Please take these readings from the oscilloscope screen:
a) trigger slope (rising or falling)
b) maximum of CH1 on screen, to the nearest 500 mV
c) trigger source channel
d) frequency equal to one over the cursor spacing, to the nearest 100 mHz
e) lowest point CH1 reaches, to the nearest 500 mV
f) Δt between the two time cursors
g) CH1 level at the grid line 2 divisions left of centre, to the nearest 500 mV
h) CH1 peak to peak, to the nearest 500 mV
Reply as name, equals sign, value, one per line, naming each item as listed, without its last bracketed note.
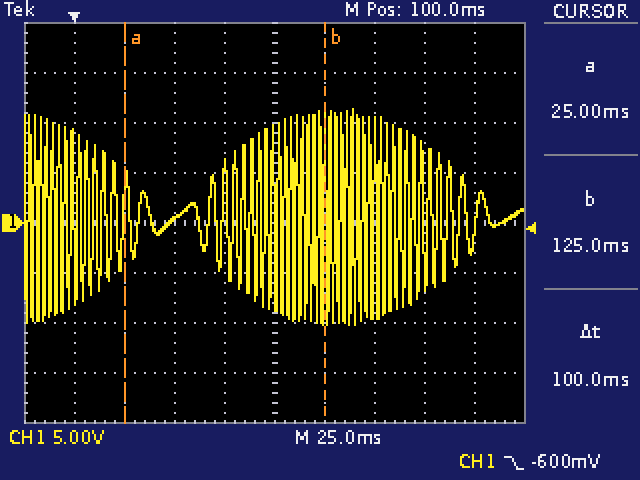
trigger slope = falling
maximum of CH1 on screen, to the nearest 500 mV = 11.5 V
trigger source channel = CH1
frequency equal to one over the cursor spacing, to the nearest 100 mHz = 10.0 Hz
lowest point CH1 reaches, to the nearest 500 mV = -10.0 V
Δt between the two time cursors = 100 ms
CH1 level at the grid line 2 divisions left of centre, to the nearest 500 mV = 500 mV
CH1 peak to peak, to the nearest 500 mV = 21.5 V
